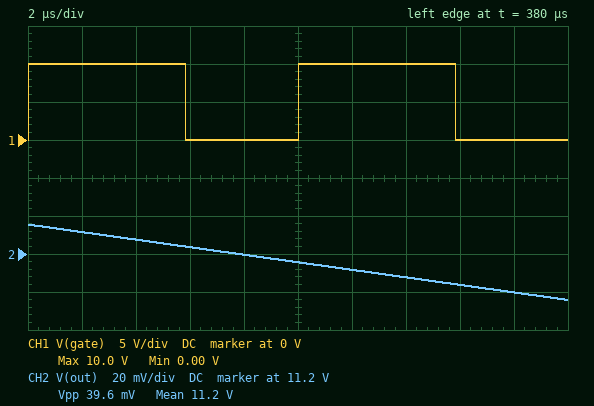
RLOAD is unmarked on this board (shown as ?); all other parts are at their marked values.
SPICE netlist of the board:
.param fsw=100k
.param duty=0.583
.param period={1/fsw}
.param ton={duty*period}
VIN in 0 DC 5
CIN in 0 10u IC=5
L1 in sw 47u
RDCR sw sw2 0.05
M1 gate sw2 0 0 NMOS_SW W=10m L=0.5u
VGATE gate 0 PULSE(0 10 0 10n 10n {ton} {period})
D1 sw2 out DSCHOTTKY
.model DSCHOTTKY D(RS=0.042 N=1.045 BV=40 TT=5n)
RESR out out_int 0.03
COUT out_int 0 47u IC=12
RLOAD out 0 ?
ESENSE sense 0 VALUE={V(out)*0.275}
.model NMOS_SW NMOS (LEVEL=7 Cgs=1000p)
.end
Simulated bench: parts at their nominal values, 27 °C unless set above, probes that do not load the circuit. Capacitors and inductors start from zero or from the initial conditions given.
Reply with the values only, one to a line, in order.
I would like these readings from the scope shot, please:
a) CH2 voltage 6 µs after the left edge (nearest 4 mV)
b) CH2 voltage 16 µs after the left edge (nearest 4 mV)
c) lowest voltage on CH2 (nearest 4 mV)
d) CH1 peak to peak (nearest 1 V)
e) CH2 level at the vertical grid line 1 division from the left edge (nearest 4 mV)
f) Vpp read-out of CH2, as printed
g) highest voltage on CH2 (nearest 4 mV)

11.204 V
11.184 V
11.176 V
10 V
11.212 V
39.6 mV
11.216 V
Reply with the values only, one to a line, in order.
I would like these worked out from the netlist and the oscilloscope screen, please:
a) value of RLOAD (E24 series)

120 Ω
